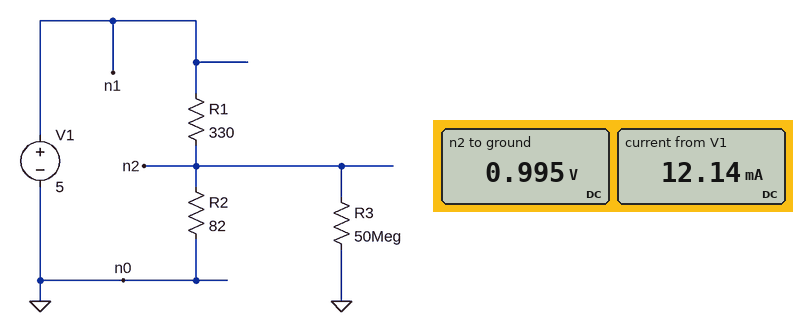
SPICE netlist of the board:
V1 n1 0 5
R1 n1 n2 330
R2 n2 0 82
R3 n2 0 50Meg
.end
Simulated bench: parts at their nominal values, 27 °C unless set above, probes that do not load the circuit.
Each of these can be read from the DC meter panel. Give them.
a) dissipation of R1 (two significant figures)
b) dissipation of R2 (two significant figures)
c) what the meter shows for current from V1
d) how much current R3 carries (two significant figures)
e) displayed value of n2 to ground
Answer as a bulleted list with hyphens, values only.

- 49 mW
- 12 mW
- 12.14 mA
- 20 nA
- 0.995 V
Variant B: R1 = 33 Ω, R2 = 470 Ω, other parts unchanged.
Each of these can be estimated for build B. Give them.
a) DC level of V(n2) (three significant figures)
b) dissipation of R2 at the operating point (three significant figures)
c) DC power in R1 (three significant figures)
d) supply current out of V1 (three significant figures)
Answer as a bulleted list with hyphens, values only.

- 4.67 V
- 46.4 mW
- 3.26 mW
- 9.94 mA
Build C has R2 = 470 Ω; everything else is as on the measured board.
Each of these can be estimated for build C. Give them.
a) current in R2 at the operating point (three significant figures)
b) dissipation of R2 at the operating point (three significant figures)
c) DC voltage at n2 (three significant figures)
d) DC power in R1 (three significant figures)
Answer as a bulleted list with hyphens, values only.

- 6.25 mA
- 18.4 mW
- 2.94 V
- 12.9 mW
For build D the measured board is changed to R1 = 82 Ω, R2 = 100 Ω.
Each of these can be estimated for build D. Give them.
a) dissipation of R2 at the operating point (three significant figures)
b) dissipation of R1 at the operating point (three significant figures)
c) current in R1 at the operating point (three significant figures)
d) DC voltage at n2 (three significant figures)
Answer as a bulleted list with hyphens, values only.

- 75.5 mW
- 61.9 mW
- 27.5 mA
- 2.75 V
